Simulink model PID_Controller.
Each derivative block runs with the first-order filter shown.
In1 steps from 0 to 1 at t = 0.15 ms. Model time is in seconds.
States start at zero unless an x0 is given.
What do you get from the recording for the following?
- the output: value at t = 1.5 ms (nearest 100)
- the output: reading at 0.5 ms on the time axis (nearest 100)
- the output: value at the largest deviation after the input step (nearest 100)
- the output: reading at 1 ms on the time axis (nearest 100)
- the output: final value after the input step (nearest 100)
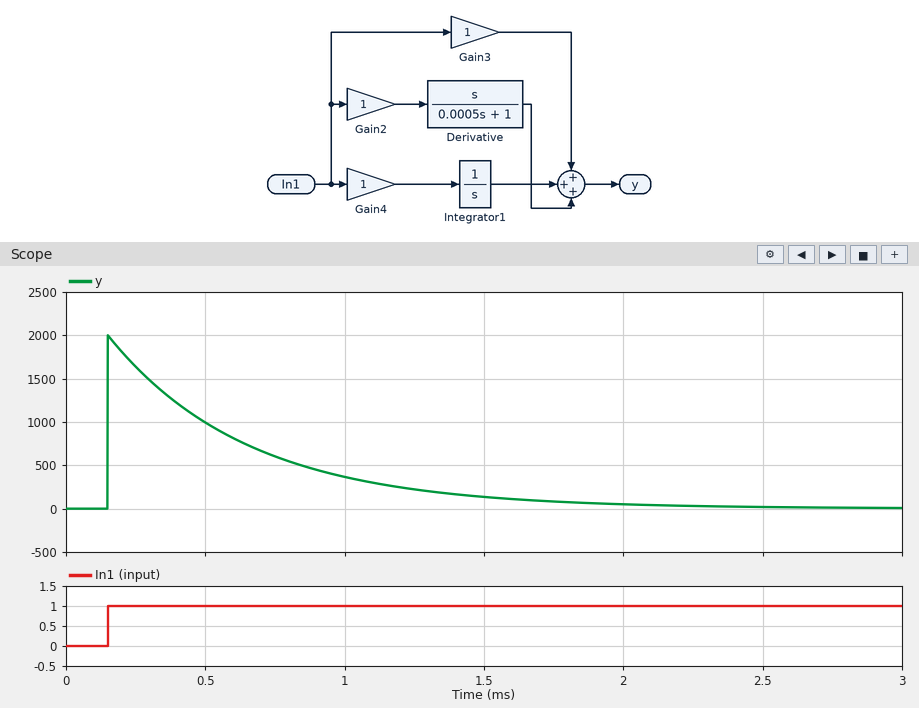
100
1000
2000
400
0
